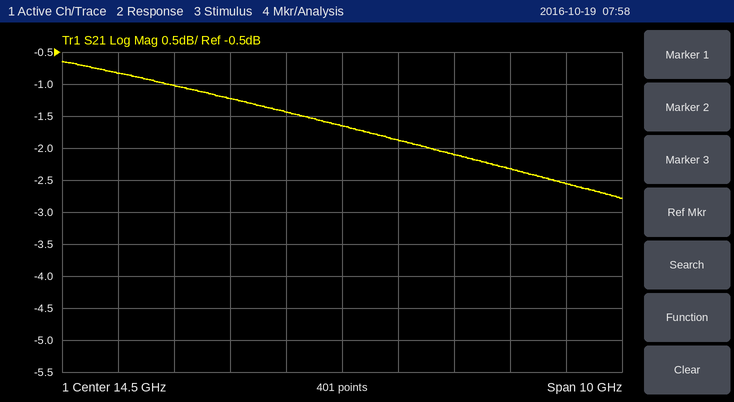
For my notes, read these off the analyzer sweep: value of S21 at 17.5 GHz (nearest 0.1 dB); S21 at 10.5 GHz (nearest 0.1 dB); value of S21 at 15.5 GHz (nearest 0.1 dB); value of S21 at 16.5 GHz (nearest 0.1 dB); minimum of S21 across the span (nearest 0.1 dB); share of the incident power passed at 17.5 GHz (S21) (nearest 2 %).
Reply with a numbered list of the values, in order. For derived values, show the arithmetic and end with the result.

1. -2.3 dB
2. -0.8 dB
3. -1.9 dB
4. -2.1 dB
5. -2.8 dB
6. 10^(-2.3/10) ≈ 58.9 %, so 58 % to the nearest 2 %
